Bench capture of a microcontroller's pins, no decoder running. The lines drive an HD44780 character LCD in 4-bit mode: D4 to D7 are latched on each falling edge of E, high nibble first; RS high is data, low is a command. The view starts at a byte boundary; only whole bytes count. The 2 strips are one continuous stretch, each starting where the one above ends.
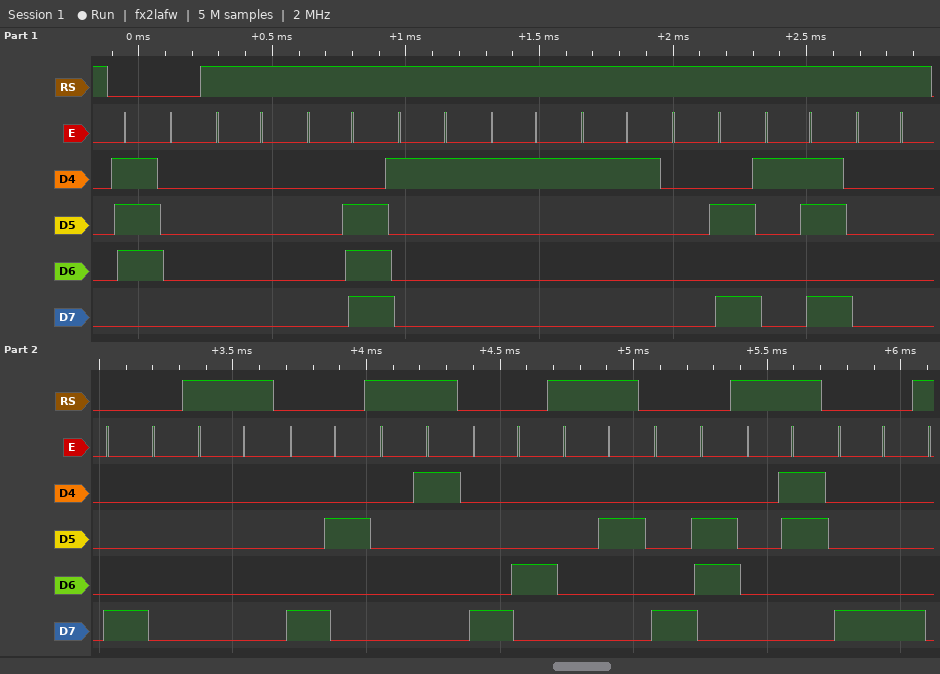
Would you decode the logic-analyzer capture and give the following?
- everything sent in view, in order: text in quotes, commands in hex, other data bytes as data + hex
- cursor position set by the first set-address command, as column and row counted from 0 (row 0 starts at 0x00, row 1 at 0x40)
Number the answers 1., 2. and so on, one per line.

1. 0x70 data 00 0E 11 11 11 0A 1B 00 0x80 data 00 0x82 data 01 0x84 data 02 0x86 data 03 0x88
2. column 0, row 0
